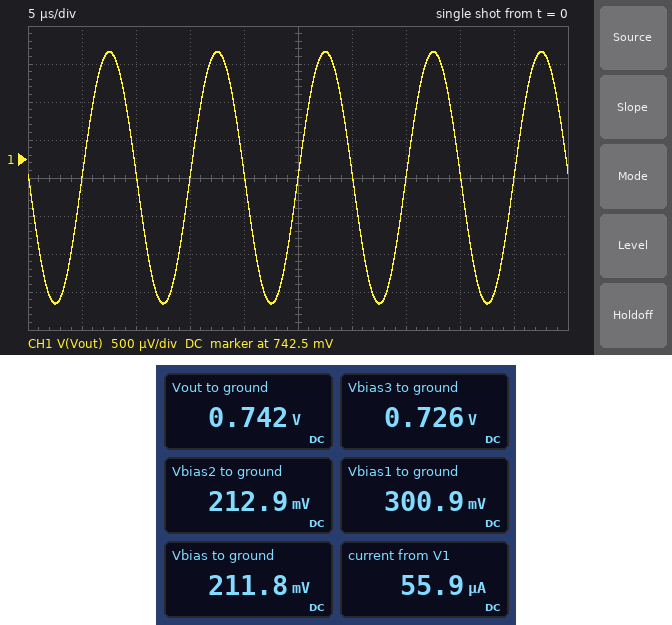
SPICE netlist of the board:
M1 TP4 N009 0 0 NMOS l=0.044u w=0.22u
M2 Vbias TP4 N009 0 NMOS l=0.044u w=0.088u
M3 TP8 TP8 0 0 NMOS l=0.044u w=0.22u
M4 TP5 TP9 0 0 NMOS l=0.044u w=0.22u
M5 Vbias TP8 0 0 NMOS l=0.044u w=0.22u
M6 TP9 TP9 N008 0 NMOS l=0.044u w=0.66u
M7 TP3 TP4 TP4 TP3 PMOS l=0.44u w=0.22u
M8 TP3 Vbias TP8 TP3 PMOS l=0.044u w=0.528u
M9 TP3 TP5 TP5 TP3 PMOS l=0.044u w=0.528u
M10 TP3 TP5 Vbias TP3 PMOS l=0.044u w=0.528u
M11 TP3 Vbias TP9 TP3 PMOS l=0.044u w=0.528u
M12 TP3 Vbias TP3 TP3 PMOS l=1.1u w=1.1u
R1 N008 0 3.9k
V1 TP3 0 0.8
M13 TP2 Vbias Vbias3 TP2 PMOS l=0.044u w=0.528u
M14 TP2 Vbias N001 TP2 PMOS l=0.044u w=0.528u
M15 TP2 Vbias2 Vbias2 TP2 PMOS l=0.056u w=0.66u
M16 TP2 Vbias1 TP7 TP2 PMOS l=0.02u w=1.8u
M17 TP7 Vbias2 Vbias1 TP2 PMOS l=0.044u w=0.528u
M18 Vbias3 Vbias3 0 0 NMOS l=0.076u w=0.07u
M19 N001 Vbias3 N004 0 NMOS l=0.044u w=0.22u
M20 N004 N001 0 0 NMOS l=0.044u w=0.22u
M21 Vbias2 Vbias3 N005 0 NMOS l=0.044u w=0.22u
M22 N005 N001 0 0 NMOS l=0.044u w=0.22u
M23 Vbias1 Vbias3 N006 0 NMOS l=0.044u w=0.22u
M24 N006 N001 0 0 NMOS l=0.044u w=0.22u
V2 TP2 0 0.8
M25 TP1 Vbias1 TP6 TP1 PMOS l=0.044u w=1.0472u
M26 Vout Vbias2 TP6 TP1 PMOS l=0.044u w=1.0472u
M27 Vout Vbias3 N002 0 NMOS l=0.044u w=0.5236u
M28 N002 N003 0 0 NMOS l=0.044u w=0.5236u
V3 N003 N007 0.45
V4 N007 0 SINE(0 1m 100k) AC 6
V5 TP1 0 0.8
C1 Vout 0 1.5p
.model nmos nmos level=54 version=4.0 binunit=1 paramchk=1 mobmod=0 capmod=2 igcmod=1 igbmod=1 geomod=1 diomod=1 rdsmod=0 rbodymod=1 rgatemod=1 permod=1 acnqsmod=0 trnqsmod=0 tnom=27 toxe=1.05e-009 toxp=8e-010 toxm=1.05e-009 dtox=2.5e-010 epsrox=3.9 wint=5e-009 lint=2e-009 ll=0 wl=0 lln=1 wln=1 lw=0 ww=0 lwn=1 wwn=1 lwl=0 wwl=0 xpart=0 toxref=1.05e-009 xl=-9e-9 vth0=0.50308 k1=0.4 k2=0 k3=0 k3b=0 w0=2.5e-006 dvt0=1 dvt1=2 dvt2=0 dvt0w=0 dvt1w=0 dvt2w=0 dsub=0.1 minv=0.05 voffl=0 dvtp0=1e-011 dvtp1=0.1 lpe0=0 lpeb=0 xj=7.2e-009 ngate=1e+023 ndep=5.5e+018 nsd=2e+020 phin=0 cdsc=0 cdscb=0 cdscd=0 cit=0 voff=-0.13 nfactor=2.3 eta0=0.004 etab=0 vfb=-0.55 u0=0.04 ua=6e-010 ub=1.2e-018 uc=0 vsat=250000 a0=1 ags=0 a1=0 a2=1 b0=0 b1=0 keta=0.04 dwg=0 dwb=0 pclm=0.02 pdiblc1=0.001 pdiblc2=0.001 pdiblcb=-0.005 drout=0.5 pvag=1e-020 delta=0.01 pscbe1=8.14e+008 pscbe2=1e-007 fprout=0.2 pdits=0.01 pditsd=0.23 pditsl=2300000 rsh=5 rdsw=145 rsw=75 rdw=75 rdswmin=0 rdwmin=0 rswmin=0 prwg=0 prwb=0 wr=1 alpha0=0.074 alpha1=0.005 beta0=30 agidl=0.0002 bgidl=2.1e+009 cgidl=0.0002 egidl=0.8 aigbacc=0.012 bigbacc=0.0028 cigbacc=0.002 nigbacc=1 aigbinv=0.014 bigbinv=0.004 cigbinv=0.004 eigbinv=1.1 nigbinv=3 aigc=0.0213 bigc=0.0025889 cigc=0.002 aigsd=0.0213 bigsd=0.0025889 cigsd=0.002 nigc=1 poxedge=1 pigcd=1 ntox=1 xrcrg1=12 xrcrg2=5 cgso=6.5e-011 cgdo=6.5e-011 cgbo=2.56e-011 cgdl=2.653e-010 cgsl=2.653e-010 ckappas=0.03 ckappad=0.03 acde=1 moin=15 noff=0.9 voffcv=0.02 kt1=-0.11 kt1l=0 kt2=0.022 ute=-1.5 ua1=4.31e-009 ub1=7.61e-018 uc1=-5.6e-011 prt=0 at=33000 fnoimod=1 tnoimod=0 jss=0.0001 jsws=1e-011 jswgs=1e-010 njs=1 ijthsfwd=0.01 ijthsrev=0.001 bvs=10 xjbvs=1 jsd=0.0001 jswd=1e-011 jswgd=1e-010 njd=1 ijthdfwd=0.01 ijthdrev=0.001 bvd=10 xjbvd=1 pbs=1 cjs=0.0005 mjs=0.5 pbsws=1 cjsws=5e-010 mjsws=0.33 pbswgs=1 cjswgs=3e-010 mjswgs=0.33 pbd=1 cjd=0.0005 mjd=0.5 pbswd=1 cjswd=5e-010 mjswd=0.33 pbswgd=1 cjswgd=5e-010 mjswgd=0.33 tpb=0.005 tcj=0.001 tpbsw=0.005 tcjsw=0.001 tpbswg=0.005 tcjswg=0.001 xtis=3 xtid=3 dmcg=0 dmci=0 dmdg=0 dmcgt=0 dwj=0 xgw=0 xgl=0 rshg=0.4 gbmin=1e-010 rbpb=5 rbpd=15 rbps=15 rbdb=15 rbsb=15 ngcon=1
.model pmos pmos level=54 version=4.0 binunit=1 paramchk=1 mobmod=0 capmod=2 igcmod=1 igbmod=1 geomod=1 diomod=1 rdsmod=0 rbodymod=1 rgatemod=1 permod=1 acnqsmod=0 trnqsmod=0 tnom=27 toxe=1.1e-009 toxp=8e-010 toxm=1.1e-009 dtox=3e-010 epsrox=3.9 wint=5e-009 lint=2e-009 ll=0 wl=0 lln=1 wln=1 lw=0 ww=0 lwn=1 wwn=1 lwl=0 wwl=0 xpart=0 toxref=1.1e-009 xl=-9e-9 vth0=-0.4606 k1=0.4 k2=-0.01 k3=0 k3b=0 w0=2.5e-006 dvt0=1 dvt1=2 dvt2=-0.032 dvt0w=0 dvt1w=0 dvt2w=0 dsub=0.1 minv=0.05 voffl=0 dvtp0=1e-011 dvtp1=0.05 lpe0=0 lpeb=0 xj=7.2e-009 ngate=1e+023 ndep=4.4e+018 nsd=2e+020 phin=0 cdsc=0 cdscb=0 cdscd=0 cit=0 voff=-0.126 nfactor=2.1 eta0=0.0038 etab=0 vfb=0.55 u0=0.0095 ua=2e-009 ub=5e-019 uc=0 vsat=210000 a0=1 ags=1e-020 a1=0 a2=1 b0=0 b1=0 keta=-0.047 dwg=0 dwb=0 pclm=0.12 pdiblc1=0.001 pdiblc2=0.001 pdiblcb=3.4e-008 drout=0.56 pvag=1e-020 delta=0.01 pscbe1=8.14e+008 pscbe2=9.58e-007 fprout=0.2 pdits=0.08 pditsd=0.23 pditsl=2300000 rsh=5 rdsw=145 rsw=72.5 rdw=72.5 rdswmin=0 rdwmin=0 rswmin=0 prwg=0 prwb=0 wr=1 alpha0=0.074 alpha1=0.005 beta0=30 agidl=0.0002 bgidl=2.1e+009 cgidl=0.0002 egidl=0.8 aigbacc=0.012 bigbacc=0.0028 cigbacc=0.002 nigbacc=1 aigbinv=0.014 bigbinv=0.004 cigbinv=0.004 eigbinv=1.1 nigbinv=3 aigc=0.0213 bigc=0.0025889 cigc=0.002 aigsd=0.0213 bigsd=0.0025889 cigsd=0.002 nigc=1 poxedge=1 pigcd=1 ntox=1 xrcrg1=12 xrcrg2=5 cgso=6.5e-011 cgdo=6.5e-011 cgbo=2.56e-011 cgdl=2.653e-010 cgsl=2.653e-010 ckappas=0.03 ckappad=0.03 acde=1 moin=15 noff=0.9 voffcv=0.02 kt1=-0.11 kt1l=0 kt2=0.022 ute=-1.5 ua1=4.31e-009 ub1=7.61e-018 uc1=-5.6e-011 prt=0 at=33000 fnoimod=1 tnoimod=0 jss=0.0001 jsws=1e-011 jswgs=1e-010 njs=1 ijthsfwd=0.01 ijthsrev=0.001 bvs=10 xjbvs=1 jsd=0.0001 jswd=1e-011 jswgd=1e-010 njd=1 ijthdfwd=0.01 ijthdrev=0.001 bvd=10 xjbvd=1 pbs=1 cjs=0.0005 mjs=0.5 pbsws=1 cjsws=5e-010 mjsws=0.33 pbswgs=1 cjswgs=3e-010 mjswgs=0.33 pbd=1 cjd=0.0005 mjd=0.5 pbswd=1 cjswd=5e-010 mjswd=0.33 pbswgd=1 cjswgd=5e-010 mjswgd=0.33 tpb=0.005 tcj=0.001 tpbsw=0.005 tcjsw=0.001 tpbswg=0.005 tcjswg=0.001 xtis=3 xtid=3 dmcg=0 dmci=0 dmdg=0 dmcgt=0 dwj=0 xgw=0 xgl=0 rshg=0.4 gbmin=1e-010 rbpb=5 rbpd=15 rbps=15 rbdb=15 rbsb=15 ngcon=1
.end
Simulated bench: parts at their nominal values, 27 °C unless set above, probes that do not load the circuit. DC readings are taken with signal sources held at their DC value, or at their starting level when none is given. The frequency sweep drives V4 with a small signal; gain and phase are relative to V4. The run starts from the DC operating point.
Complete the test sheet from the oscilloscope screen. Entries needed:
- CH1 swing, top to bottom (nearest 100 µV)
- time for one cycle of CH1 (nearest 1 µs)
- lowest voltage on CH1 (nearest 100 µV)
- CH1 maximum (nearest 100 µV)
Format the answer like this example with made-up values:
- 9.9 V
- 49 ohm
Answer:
- 3.3 mV
- 10 µs
- 740.6 mV
- 743.9 mV
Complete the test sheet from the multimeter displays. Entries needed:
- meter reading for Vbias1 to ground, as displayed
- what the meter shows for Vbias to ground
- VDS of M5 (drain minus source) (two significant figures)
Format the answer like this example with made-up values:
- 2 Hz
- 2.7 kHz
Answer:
- 300.9 mV
- 211.8 mV
- 210 mV
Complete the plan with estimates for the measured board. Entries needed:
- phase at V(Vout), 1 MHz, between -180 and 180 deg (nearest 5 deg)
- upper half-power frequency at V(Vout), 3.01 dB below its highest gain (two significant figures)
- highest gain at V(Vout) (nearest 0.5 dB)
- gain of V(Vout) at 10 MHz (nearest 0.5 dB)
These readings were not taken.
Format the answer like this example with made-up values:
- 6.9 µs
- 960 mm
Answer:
- 170 deg
- 5.2 MHz
- 4.5 dB
- -2.5 dB
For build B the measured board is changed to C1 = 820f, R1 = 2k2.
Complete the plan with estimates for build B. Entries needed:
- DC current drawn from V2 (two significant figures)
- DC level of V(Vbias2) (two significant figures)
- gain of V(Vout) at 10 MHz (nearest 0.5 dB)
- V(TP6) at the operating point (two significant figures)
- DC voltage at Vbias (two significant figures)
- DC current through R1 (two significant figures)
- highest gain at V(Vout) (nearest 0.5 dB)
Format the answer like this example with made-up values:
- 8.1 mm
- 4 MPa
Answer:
- 81 µA
- 170 mV
- -6.0 dB
- 790 mV
- 130 mV
- 29 µA
- -5.5 dB
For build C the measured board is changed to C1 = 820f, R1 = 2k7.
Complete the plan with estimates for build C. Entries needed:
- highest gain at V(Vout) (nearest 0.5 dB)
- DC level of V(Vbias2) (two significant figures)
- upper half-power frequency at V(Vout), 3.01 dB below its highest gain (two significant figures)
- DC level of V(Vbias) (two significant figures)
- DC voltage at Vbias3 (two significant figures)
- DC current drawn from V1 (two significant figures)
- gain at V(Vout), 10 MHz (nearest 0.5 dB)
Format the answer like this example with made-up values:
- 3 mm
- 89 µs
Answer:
- -4.5 dB
- 180 mV
- 27 MHz
- 160 mV
- 750 mV
- 88 µA
- -5.0 dB
